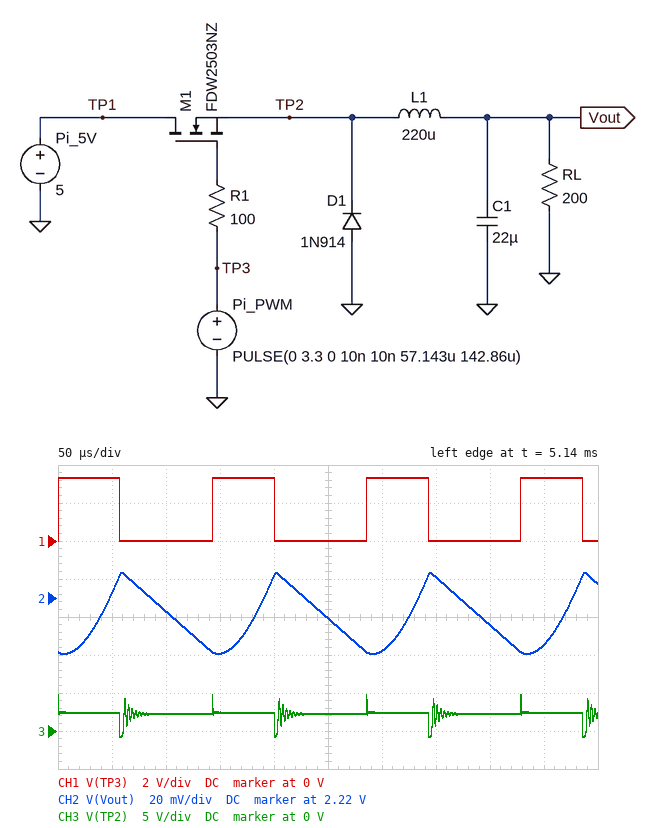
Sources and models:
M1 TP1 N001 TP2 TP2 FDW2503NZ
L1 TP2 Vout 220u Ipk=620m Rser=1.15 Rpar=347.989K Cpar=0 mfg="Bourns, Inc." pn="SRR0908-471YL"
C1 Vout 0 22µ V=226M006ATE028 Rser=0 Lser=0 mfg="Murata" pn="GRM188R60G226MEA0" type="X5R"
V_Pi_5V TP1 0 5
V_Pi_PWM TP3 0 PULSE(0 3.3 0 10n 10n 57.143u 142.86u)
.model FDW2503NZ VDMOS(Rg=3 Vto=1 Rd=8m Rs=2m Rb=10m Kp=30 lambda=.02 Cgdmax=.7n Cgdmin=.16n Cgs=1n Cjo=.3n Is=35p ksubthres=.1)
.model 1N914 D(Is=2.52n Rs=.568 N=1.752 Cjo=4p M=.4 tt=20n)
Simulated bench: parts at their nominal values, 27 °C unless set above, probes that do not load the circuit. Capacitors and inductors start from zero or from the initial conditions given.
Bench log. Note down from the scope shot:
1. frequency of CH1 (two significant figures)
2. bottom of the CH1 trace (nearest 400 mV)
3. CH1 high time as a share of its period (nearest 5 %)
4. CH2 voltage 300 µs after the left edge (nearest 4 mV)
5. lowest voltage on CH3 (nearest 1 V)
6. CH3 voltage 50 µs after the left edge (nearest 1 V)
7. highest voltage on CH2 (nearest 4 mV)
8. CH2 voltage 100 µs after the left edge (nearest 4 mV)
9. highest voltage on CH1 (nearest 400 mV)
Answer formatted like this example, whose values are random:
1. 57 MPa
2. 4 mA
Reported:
1. 7.0 kHz
2. 0 V
3. 40 %
4. 2.192 V
5. -1 V
6. 2 V
7. 2.232 V
8. 2.212 V
9. 3.2 V
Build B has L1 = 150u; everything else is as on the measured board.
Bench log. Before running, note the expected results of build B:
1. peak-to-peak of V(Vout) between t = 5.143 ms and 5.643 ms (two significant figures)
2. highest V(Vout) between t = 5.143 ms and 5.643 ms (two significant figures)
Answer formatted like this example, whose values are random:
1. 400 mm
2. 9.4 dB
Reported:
1. 44 mV
2. 2.3 V
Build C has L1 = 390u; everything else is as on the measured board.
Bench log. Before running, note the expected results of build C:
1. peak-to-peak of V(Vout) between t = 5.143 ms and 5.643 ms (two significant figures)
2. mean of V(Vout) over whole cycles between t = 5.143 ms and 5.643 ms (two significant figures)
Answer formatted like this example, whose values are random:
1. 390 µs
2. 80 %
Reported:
1. 40 mV
2. 2.1 V
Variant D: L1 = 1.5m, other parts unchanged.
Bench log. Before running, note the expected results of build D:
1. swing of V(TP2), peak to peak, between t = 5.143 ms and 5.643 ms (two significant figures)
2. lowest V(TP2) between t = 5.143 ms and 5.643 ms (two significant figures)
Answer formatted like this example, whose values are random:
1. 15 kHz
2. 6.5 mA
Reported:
1. 4.9 V
2. -750 mV
